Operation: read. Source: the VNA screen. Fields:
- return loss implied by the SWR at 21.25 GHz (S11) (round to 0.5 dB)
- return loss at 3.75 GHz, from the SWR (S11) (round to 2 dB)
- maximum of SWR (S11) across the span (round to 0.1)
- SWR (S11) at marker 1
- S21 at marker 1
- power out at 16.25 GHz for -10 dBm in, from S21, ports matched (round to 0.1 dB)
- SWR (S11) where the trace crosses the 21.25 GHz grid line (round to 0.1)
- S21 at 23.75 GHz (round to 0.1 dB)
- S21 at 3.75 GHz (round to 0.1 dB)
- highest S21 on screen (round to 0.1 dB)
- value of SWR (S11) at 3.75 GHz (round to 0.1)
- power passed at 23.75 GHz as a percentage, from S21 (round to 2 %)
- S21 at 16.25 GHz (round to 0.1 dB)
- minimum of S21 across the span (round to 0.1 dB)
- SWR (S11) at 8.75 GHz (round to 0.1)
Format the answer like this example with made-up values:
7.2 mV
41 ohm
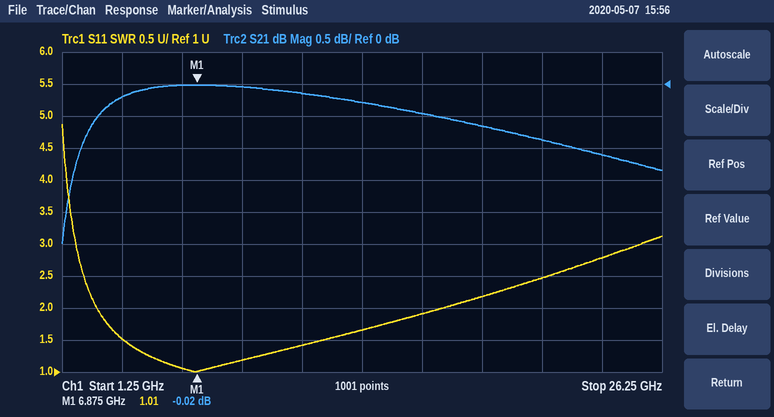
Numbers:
7.5 dB
14 dB
4.9
1.01
-0.02 dB
-10.5 dBm
2.5
-1.1 dB
-0.2 dB
0.0 dB
1.5
78 %
-0.5 dB
-2.5 dB
1.2
